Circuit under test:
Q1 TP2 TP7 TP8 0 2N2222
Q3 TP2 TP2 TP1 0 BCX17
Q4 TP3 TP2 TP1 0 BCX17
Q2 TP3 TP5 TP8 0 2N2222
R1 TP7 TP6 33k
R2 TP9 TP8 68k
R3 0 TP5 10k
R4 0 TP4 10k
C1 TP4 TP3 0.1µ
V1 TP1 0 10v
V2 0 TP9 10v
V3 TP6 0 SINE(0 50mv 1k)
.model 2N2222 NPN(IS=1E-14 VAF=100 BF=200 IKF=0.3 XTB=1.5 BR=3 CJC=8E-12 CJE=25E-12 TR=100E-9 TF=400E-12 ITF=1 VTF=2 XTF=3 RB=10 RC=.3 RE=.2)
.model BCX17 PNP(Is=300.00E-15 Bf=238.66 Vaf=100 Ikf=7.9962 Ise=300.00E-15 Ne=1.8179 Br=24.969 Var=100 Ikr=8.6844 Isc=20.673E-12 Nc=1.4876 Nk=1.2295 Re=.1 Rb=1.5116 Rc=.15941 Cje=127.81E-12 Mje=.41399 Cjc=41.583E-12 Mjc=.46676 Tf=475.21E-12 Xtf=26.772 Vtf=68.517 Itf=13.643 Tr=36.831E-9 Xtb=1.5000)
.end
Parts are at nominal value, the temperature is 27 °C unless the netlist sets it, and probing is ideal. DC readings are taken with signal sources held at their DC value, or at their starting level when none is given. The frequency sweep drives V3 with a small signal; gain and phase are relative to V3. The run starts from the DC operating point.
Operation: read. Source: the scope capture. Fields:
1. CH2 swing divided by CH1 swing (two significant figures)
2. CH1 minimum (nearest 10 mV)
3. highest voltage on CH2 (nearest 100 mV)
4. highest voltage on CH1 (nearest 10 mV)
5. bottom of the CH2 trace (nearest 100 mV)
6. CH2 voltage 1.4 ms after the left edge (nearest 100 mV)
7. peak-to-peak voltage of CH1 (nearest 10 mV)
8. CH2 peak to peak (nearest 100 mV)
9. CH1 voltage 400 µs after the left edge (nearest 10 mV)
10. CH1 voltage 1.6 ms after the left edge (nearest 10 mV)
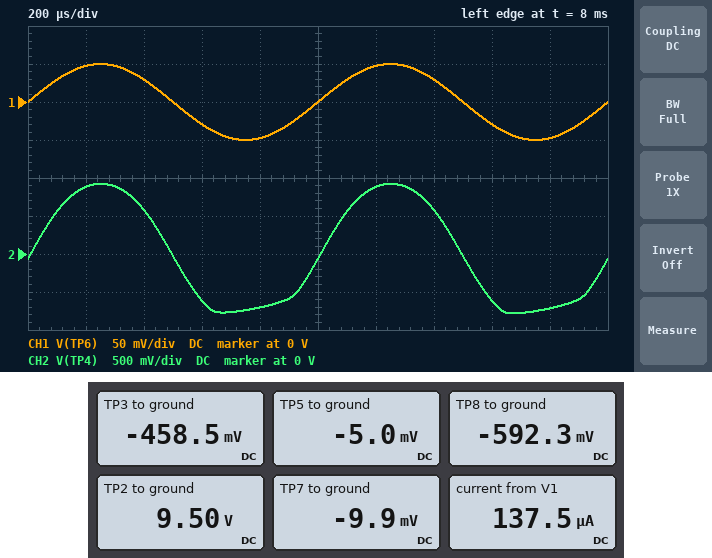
17
-50 mV
900 mV
50 mV
-800 mV
600 mV
100 mV
1.7 V
30 mV
-30 mV
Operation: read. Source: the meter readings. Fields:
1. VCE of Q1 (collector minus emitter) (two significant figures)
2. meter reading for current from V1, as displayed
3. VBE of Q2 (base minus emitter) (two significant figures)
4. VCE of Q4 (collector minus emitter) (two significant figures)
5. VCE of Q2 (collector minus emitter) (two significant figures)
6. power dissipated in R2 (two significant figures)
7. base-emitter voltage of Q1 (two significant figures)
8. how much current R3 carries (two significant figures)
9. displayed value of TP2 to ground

10 V
137.5 µA
590 mV
-10 V
130 mV
1.3 mW
580 mV
500 nA
9.50 V
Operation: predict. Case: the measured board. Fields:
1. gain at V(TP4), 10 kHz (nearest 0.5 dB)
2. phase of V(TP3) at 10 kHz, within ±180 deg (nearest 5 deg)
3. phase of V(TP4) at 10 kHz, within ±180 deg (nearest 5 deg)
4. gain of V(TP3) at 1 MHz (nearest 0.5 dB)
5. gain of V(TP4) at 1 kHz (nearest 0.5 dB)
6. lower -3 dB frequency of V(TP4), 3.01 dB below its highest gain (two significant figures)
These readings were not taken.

19.5 dB
-5 deg
-5 deg
-2.5 dB
19.5 dB
90 Hz
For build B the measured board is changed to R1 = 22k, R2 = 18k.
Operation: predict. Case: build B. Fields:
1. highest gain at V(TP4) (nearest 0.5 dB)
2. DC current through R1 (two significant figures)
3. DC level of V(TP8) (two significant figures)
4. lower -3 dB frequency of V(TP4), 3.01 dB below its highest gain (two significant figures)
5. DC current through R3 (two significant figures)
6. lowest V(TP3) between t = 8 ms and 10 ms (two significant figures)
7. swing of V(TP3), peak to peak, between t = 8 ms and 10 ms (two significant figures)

13.0 dB
1.1 µA
-640 mV
150 Hz
2.0 µA
-580 mV
3.8 V
